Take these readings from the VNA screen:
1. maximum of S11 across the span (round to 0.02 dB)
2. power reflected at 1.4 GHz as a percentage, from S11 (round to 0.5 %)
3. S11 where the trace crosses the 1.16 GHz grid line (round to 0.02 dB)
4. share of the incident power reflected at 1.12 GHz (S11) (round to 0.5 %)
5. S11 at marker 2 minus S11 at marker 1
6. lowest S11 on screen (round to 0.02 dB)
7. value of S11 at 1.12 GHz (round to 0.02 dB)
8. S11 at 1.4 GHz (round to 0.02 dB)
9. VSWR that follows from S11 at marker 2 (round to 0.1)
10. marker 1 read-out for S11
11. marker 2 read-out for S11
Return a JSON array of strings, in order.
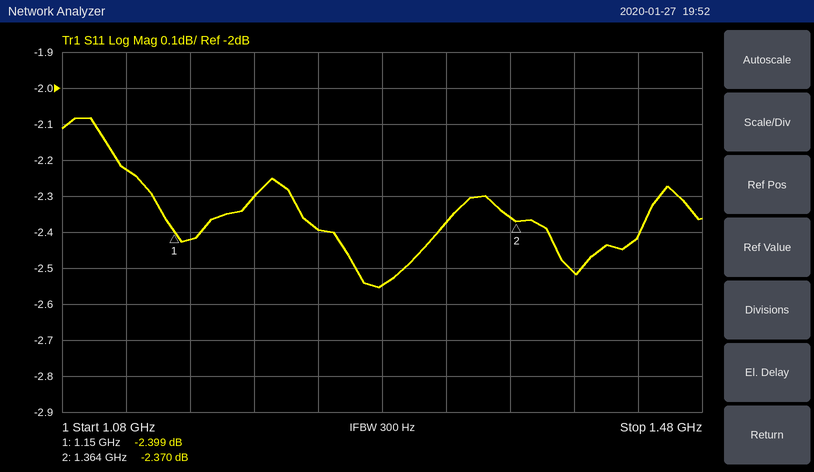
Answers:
["-2.08 dB", "56.0 %", "-2.42 dB", "60.0 %", "0.029 dB", "-2.56 dB", "-2.22 dB", "-2.52 dB", "7.4", "-2.399 dB", "-2.370 dB"]
